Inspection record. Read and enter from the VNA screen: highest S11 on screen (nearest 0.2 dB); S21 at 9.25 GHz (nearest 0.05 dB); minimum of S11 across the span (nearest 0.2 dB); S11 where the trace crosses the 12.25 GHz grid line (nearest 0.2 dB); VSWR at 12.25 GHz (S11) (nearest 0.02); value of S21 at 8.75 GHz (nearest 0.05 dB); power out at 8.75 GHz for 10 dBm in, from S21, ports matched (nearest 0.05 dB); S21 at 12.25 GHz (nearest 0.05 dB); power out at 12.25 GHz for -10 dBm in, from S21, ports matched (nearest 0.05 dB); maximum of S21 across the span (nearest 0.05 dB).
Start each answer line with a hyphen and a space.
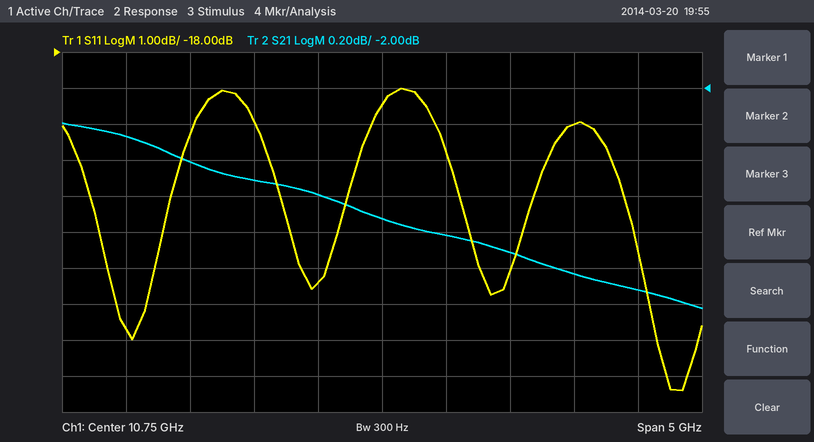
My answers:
- -19.0 dB
- -2.40 dB
- -27.4 dB
- -20.0 dB
- 1.22
- -2.25 dB
- 7.75 dBm
- -3.05 dB
- -13.05 dBm
- -2.20 dB
